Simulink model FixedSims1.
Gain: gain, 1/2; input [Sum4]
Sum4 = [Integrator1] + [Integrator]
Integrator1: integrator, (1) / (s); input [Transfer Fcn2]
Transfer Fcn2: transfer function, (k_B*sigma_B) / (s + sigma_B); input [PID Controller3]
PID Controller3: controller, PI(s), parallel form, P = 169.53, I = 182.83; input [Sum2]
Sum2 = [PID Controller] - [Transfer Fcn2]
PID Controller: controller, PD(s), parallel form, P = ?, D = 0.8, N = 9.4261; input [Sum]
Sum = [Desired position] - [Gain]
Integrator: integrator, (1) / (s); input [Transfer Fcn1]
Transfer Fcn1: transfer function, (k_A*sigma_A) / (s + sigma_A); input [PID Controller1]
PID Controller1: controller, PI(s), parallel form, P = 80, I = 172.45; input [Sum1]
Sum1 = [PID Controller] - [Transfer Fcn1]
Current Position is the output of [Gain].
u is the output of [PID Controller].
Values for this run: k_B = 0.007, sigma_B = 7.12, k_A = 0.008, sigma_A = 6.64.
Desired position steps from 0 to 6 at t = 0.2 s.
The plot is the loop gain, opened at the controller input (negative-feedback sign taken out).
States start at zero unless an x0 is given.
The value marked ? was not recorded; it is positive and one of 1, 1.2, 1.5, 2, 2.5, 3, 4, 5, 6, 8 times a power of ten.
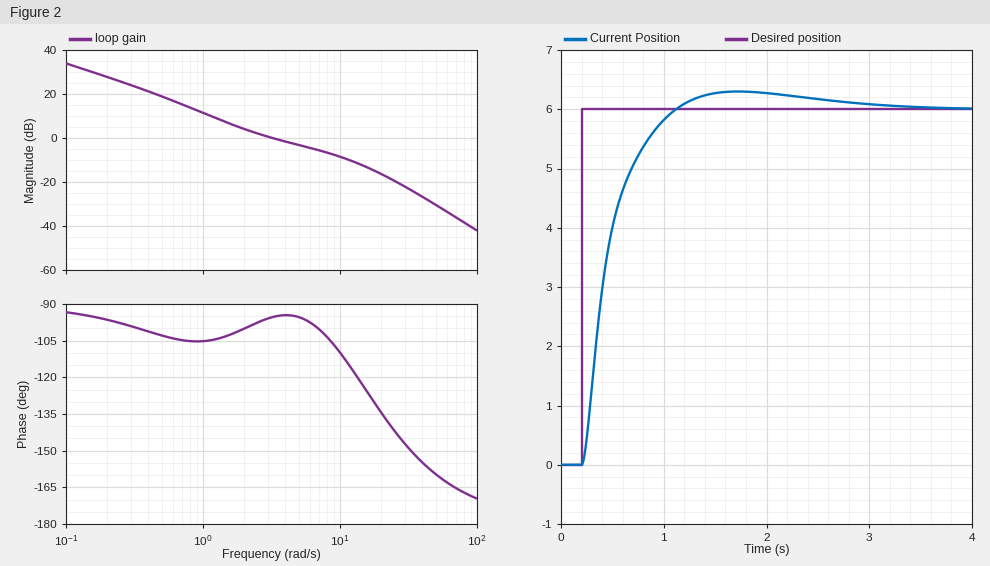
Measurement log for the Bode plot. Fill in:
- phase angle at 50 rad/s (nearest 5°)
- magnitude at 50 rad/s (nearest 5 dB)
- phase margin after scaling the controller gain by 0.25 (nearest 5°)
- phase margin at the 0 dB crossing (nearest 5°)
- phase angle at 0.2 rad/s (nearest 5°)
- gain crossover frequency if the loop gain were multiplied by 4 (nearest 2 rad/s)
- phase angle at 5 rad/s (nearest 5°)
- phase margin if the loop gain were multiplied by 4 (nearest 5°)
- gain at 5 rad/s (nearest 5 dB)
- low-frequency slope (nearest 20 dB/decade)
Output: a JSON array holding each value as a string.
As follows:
["-160°", "-30 dB", "75°", "85°", "-95°", "14 rad/s", "-95°", "60°", "-5 dB", "-20 dB/decade"]
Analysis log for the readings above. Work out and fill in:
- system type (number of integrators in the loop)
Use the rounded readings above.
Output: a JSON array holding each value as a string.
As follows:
["1"]
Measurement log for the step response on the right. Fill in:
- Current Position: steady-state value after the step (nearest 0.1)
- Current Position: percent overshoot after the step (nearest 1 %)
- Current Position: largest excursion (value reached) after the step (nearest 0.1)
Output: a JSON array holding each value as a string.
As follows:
["6.0", "5 %", "6.3"]
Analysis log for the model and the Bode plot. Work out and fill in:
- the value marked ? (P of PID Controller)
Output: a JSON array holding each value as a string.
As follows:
["5"]
